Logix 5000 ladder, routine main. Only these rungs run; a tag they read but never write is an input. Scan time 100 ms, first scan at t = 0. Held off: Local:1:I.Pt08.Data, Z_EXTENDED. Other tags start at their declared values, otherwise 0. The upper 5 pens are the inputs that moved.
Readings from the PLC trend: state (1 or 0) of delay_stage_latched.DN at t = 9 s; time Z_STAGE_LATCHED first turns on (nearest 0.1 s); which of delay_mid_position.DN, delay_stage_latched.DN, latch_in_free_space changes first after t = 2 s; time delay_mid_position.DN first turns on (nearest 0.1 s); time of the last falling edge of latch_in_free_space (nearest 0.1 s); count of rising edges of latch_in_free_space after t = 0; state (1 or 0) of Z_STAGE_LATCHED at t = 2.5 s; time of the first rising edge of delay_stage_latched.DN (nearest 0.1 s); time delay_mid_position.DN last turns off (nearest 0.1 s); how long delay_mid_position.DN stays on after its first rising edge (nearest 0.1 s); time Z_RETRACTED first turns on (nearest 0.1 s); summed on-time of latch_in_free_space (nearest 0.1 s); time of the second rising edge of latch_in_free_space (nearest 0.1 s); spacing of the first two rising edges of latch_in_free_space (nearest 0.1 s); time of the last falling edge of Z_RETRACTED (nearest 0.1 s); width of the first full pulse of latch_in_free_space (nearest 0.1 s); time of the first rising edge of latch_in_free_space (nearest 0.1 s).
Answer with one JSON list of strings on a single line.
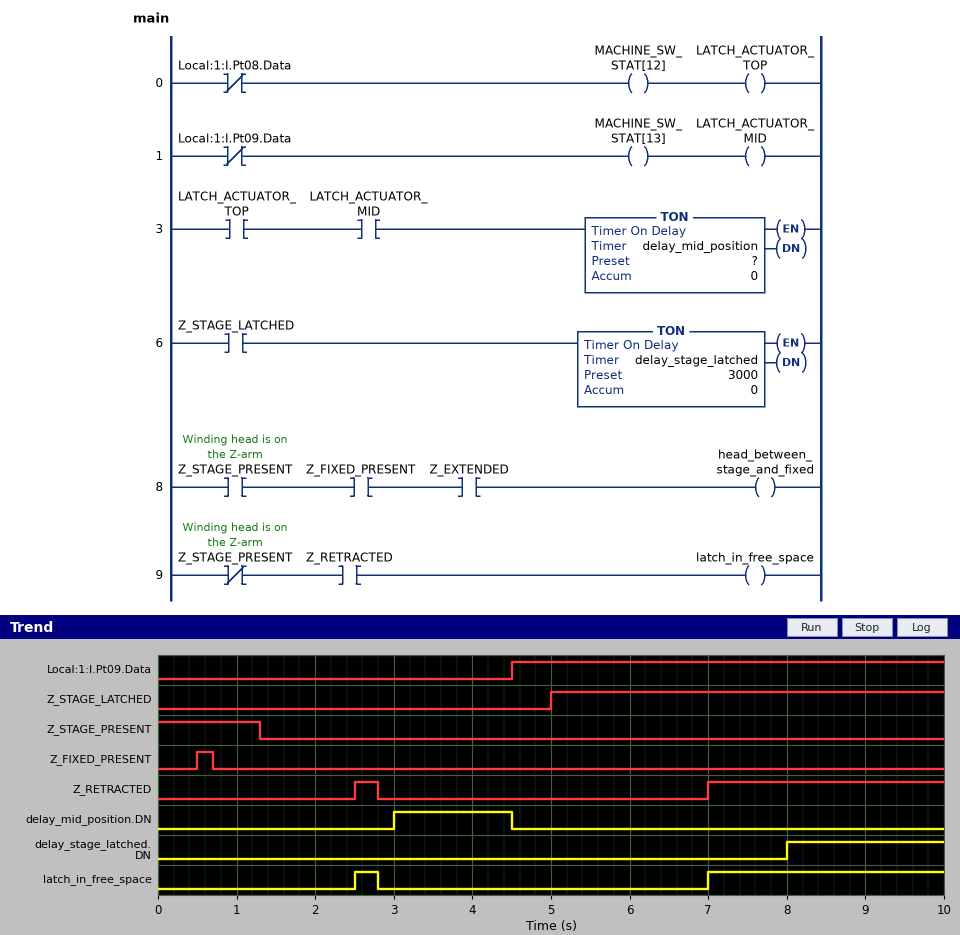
["1", "5.0 s", "latch_in_free_space", "3.0 s", "2.8 s", "2", "0", "8.0 s", "4.5 s", "1.5 s", "2.5 s", "3.3 s", "7.0 s", "4.5 s", "2.8 s", "0.3 s", "2.5 s"]
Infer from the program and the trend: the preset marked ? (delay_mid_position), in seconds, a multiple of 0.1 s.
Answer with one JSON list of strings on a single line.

["3.0 s"]
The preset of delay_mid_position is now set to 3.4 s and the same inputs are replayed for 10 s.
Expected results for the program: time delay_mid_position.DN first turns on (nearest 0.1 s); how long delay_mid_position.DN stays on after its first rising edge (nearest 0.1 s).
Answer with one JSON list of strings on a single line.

["3.4 s", "1.1 s"]
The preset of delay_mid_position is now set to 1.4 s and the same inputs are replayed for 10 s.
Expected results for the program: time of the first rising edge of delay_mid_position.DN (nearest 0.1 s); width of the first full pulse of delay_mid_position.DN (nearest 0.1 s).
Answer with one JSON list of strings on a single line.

["1.4 s", "3.1 s"]
